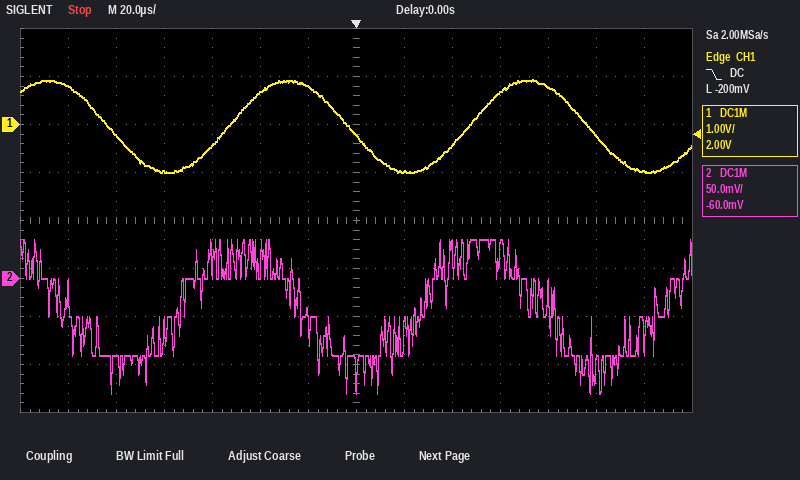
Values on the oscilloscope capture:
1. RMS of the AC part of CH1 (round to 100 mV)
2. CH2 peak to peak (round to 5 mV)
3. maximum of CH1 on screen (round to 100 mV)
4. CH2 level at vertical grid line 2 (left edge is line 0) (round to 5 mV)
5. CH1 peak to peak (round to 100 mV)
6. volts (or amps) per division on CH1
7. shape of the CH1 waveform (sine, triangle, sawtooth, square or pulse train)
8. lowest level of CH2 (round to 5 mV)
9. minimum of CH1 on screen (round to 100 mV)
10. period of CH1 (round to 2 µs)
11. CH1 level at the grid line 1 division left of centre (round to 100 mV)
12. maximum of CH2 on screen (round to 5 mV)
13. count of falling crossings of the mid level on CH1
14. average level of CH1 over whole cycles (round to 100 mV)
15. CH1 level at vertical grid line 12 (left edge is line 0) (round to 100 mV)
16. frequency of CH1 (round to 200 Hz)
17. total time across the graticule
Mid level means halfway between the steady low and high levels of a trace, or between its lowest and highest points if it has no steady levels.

700 mV
160 mV
900 mV
-80 mV
1.9 V
1 V
sine
-120 mV
-1.0 V
100 µs
800 mV
40 mV
3
0.0 V
-200 mV
10.0 kHz
280 µs
